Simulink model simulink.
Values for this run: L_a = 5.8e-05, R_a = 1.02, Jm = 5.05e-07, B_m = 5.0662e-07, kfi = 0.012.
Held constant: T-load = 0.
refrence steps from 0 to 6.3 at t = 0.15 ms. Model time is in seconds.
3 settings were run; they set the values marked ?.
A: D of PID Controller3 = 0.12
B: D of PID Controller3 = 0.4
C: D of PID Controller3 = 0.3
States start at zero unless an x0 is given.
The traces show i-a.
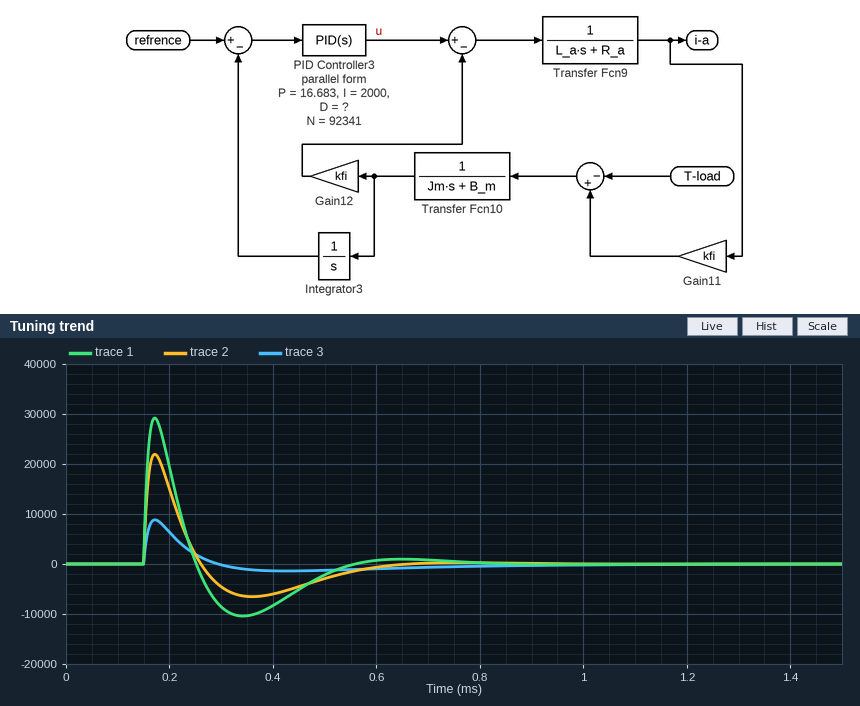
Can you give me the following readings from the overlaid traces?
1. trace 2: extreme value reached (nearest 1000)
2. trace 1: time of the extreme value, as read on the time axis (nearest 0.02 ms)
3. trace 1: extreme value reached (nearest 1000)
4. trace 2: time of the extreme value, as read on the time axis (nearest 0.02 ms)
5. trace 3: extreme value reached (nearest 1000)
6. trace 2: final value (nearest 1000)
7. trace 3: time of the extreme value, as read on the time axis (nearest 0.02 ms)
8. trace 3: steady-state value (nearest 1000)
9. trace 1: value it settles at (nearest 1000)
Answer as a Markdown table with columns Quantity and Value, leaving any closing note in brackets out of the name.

| Quantity | Value |
|---|---|
| trace 2: extreme value reached | 22000 |
| trace 1: time of the extreme value, as read on the time axis | 0.18 ms |
| trace 1: extreme value reached | 29000 |
| trace 2: time of the extreme value, as read on the time axis | 0.18 ms |
| trace 3: extreme value reached | 9000 |
| trace 2: final value | 0 |
| trace 3: time of the extreme value, as read on the time axis | 0.18 ms |
| trace 3: steady-state value | 0 |
| trace 1: value it settles at | 0 |
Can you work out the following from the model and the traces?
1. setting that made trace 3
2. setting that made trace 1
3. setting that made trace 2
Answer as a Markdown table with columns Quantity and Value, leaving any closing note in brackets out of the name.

| Quantity | Value |
|---|---|
| setting that made trace 3 | A |
| setting that made trace 1 | B |
| setting that made trace 2 | C |
